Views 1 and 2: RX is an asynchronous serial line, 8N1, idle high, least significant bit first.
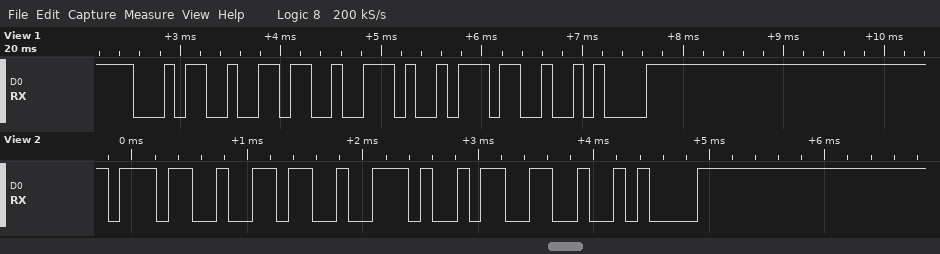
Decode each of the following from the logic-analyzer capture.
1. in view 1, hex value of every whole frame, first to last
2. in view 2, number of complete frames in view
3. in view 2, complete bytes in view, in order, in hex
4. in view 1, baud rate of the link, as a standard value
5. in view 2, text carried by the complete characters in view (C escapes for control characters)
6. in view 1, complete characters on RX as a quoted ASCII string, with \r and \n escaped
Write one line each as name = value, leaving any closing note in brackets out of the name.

in view 1, hex value of every whole frame, first to last = 34 36 2E 37 0A
in view 2, number of complete frames in view = 5
in view 2, complete bytes in view, in order, in hex = 37 36 2E 33 0A
in view 1, baud rate of the link, as a standard value = 9600 baud
in view 2, text carried by the complete characters in view = "76.3\n"
in view 1, complete characters on RX as a quoted ASCII string, with \r and \n escaped = "46.7\n"
